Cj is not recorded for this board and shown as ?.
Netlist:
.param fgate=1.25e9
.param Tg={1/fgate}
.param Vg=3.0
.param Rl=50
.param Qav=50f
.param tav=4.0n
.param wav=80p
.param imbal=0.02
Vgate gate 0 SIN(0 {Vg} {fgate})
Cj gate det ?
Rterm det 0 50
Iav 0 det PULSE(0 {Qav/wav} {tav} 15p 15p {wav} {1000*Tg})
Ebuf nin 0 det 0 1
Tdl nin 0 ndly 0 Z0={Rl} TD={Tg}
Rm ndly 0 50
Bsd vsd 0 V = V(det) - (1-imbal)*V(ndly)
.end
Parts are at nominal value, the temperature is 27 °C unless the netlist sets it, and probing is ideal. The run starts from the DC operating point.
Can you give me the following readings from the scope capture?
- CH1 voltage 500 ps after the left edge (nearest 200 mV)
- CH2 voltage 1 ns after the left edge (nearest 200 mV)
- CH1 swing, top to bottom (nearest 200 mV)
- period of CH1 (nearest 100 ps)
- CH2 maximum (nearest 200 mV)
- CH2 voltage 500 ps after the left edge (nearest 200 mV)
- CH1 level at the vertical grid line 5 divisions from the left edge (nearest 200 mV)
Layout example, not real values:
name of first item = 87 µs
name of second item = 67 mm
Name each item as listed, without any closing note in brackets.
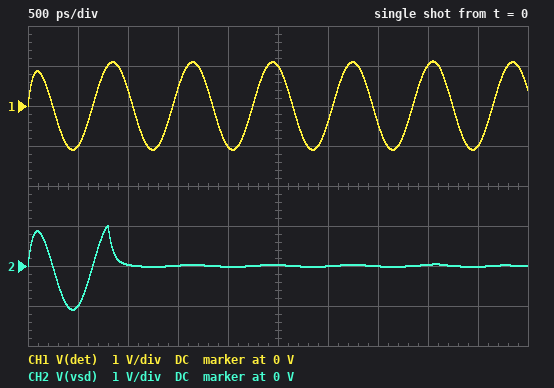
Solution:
CH1 voltage 500 ps after the left edge = -1.0 V
CH2 voltage 1 ns after the left edge = 0 V
CH1 swing, top to bottom = 2.2 V
period of CH1 = 800 ps
CH2 maximum = 1.0 V
CH2 voltage 500 ps after the left edge = -1.0 V
CH1 level at the vertical grid line 5 divisions from the left edge = 1.0 V
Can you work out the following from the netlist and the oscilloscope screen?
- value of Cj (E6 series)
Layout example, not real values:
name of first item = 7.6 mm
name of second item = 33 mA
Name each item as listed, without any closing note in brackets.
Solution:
value of Cj = 1 pF
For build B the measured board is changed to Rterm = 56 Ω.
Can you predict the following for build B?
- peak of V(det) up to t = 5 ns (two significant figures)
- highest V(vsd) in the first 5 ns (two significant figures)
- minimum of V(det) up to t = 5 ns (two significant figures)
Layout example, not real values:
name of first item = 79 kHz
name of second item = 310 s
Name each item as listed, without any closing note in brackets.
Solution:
peak of V(det) up to t = 5 ns = 1.2 V
highest V(vsd) in the first 5 ns = 1.1 V
minimum of V(det) up to t = 5 ns = -1.2 V
